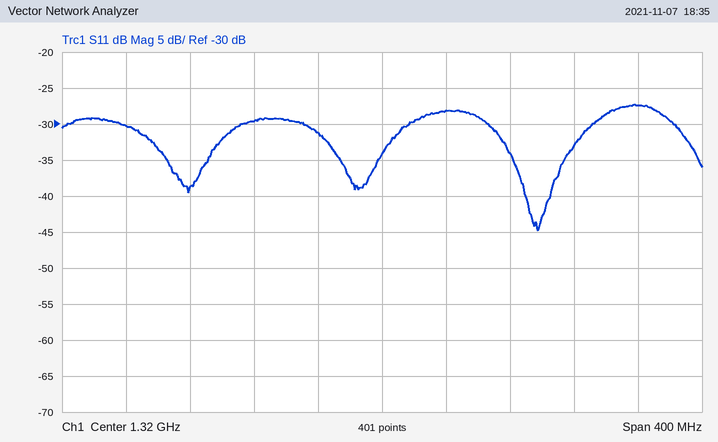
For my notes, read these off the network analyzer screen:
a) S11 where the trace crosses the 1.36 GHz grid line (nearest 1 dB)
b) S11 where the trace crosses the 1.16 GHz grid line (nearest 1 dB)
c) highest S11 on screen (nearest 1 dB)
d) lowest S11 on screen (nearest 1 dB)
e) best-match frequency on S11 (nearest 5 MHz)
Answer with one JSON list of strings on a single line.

["-28 dB", "-30 dB", "-27 dB", "-45 dB", "1.415 GHz"]
